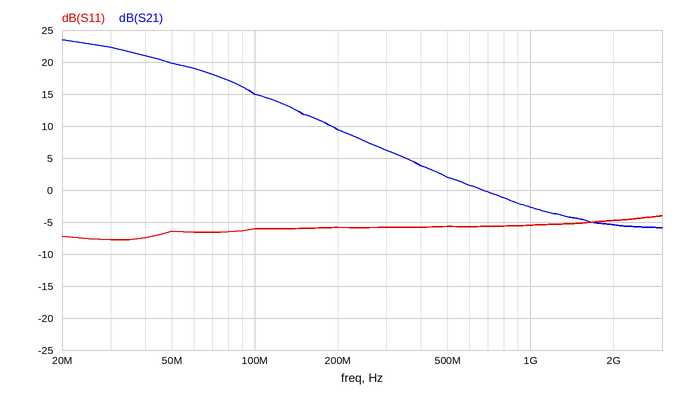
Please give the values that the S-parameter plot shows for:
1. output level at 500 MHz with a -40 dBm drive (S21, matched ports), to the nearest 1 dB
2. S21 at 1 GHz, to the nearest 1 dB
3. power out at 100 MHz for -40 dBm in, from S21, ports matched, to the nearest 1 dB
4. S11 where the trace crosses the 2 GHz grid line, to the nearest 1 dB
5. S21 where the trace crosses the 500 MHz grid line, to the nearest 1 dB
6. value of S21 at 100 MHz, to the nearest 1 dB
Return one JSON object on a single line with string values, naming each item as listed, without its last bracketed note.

{"output level at 500 MHz with a -40 dBm drive (S21, matched ports), to the nearest 1 dB": "-38 dBm", "S21 at 1 GHz, to the nearest 1 dB": "-3 dB", "power out at 100 MHz for -40 dBm in, from S21, ports matched, to the nearest 1 dB": "-25 dBm", "S11 where the trace crosses the 2 GHz grid line, to the nearest 1 dB": "-5 dB", "S21 where the trace crosses the 500 MHz grid line, to the nearest 1 dB": "2 dB", "value of S21 at 100 MHz, to the nearest 1 dB": "15 dB"}
